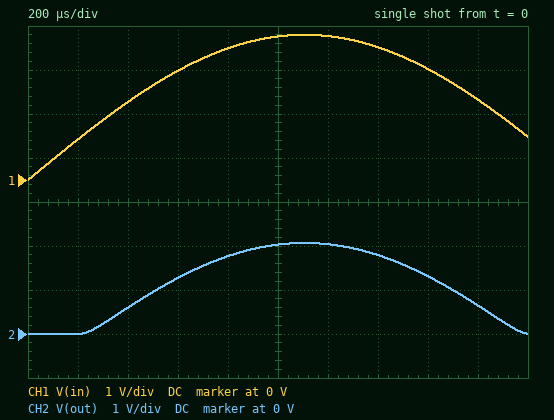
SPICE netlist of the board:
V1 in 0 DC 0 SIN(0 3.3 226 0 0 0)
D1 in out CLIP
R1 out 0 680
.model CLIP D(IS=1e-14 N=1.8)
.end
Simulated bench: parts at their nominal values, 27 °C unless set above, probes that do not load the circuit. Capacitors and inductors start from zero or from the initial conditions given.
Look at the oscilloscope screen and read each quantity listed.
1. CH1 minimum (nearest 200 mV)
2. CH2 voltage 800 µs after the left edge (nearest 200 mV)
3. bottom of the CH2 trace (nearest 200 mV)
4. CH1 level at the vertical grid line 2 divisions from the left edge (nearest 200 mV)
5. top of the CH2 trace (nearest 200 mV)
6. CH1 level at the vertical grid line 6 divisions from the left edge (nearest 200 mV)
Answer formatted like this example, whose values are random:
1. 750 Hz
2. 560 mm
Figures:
1. 0 V
2. 1.8 V
3. 0 V
4. 1.8 V
5. 2.0 V
6. 3.2 V
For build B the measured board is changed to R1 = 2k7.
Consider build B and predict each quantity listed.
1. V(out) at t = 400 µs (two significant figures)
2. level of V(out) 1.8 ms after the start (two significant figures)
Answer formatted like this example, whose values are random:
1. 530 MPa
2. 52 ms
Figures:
1. 660 mV
2. 710 mV
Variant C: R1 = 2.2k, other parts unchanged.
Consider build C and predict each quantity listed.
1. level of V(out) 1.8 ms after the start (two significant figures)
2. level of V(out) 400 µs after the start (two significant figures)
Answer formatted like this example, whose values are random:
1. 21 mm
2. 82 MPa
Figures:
1. 700 mV
2. 650 mV
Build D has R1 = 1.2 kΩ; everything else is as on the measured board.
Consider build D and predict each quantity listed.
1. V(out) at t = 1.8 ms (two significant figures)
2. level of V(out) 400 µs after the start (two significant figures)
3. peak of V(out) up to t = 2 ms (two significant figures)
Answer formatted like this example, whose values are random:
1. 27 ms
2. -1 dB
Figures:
1. 670 mV
2. 630 mV
3. 2.1 V
